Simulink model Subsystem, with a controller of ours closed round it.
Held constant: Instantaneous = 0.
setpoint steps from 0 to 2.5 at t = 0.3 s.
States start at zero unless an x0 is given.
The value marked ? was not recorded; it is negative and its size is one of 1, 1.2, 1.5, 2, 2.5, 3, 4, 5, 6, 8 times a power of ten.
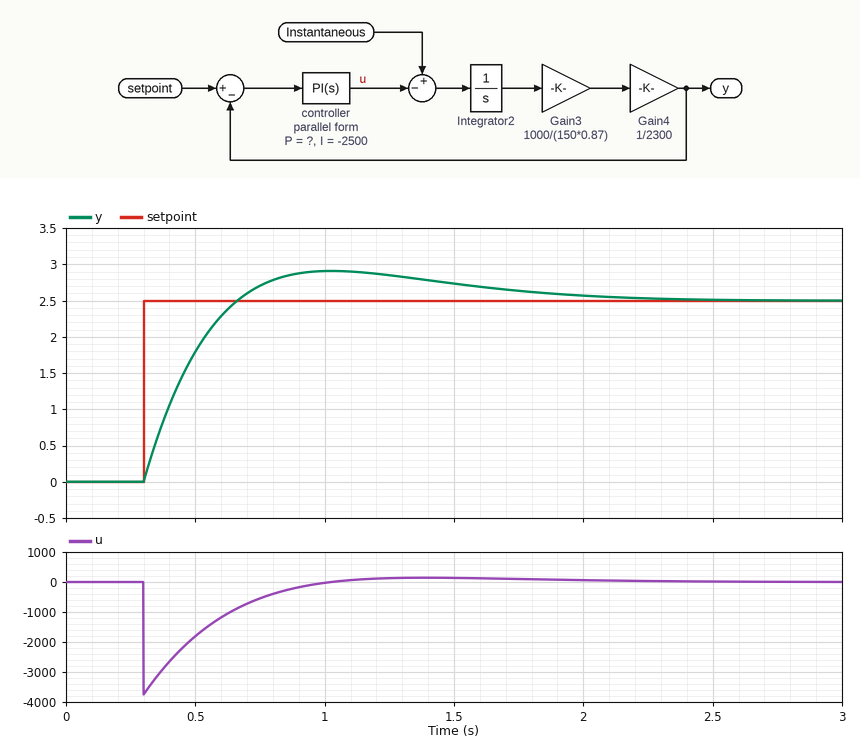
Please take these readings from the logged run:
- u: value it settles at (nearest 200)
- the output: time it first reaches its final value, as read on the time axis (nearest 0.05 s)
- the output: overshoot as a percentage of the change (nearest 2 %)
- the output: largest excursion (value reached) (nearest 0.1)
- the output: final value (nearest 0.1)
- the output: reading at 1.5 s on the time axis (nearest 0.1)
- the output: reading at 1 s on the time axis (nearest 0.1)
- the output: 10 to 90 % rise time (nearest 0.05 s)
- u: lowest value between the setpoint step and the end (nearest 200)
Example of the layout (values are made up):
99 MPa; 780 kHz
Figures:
0; 0.65 s; 16 %; 2.9; 2.5; 2.7; 2.9; 0.25 s; -3800
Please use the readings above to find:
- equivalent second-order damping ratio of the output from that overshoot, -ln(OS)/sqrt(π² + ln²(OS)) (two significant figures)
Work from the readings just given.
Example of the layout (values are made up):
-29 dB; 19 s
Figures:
0.50
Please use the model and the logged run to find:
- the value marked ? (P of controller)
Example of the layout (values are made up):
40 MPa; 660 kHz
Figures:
-1500
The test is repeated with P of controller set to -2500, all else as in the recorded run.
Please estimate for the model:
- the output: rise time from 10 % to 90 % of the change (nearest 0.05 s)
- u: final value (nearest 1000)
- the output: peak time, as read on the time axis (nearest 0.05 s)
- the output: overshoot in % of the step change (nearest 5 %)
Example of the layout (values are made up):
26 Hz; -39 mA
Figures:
0.20 s; 0; 0.90 s; 10 %
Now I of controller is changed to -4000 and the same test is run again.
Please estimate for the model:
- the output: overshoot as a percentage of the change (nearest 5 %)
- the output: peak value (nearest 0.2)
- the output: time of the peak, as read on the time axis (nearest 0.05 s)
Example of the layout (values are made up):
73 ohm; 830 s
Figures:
20 %; 3.0; 0.90 s
